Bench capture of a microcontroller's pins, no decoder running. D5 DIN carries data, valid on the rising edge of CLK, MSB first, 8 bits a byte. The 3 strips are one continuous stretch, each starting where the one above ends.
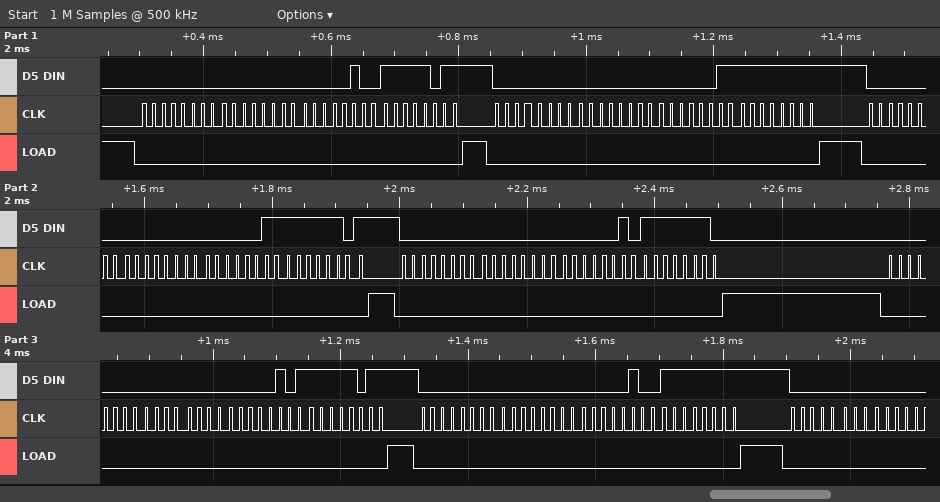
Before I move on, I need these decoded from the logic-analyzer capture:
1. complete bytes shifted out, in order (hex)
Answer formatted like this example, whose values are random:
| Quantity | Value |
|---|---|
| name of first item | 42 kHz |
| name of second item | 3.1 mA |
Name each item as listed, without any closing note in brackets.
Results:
| Quantity | Value |
|---|---|
| complete bytes shifted out, in order | 00 00 04 FB 00 00 03 FF 00 00 03 FD 00 00 02 FE 00 00 05 FB 00 00 04 FF 00 |
